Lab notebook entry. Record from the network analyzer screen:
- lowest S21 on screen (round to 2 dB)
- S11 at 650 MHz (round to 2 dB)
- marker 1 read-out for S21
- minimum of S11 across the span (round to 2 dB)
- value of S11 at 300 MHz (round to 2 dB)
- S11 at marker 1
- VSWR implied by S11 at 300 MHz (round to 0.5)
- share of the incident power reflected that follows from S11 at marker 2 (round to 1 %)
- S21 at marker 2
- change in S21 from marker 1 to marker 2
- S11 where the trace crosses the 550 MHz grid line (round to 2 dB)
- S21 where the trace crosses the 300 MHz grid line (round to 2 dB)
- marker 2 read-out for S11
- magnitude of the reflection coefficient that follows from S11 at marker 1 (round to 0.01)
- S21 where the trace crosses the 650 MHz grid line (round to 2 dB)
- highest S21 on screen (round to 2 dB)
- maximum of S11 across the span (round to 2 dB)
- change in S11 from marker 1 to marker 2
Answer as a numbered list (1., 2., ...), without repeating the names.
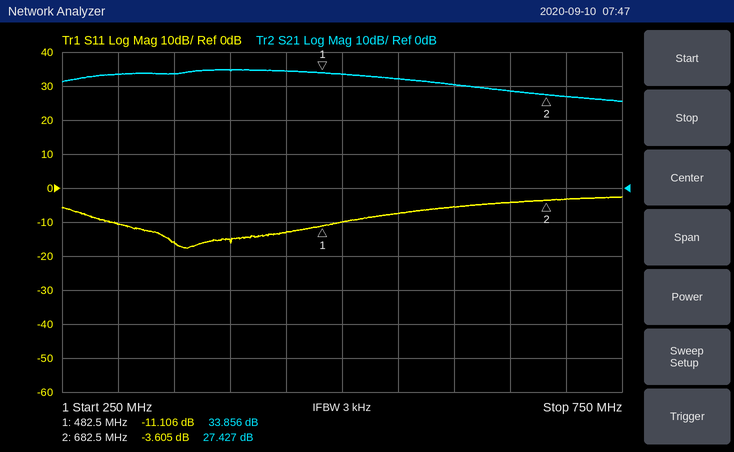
1. 26 dB
2. -4 dB
3. 33.856 dB
4. -18 dB
5. -10 dB
6. -11.106 dB
7. 2.0
8. 44 %
9. 27.427 dB
10. -6.429 dB
11. -8 dB
12. 34 dB
13. -3.605 dB
14. 0.28
15. 28 dB
16. 34 dB
17. -2 dB
18. 7.501 dB
